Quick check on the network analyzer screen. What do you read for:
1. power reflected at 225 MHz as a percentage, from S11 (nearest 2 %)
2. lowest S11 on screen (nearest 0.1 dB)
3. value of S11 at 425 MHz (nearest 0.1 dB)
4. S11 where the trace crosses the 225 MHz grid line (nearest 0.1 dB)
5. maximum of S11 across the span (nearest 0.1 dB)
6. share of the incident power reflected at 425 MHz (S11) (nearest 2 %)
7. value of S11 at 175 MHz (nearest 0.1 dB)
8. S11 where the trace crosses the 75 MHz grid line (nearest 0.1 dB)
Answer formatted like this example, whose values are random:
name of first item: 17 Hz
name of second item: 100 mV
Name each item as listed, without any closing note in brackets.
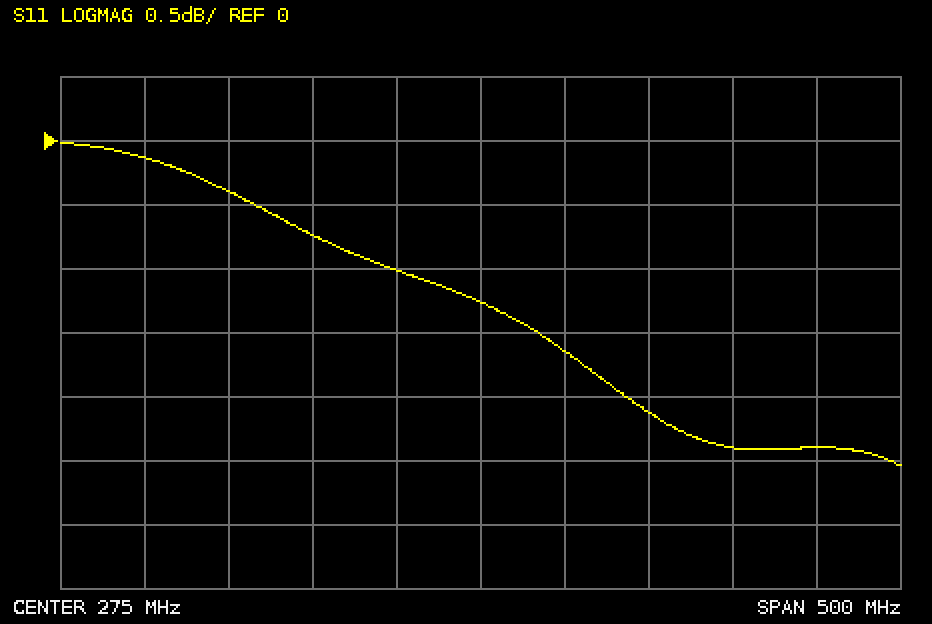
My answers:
power reflected at 225 MHz as a percentage, from S11: 80 %
lowest S11 on screen: -2.5 dB
value of S11 at 425 MHz: -2.4 dB
S11 where the trace crosses the 225 MHz grid line: -1.0 dB
maximum of S11 across the span: 0.0 dB
share of the incident power reflected at 425 MHz (S11): 58 %
value of S11 at 175 MHz: -0.7 dB
S11 where the trace crosses the 75 MHz grid line: -0.1 dB
